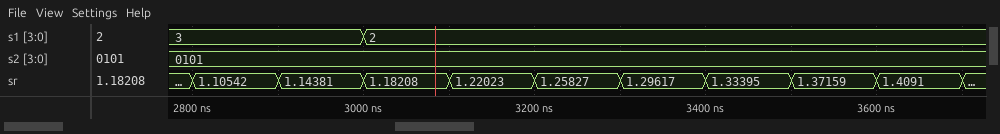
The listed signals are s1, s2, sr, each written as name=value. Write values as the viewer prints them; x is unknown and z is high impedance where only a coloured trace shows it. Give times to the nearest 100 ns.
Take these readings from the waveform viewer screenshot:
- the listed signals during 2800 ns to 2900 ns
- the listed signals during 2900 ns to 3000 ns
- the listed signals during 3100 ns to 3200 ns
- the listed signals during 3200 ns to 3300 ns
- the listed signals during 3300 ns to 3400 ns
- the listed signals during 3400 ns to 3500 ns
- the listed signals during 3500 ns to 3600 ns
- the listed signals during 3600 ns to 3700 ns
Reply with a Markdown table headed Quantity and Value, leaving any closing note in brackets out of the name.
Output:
| Quantity | Value |
|---|---|
| the listed signals during 2800 ns to 2900 ns | s1=3, s2=0101, sr=1.10542 |
| the listed signals during 2900 ns to 3000 ns | s1=3, s2=0101, sr=1.14381 |
| the listed signals during 3100 ns to 3200 ns | s1=2, s2=0101, sr=1.22023 |
| the listed signals during 3200 ns to 3300 ns | s1=2, s2=0101, sr=1.25827 |
| the listed signals during 3300 ns to 3400 ns | s1=2, s2=0101, sr=1.29617 |
| the listed signals during 3400 ns to 3500 ns | s1=2, s2=0101, sr=1.33395 |
| the listed signals during 3500 ns to 3600 ns | s1=2, s2=0101, sr=1.37159 |
| the listed signals during 3600 ns to 3700 ns | s1=2, s2=0101, sr=1.4091 |
